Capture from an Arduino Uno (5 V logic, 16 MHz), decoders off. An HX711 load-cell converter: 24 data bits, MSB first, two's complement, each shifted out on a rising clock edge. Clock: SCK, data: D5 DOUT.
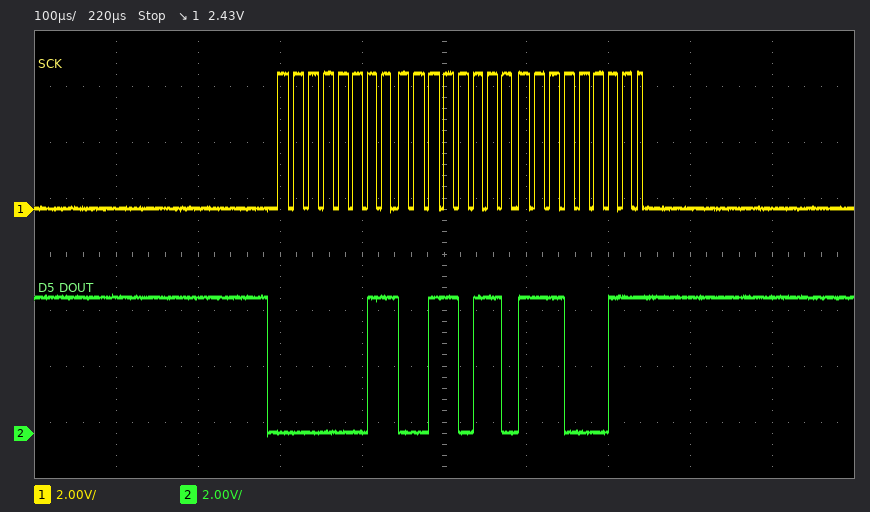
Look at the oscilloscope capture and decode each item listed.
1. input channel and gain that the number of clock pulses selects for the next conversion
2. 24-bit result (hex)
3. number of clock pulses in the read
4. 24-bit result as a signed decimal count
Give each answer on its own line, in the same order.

channel A, gain 128
0x0336E3
25
210659
